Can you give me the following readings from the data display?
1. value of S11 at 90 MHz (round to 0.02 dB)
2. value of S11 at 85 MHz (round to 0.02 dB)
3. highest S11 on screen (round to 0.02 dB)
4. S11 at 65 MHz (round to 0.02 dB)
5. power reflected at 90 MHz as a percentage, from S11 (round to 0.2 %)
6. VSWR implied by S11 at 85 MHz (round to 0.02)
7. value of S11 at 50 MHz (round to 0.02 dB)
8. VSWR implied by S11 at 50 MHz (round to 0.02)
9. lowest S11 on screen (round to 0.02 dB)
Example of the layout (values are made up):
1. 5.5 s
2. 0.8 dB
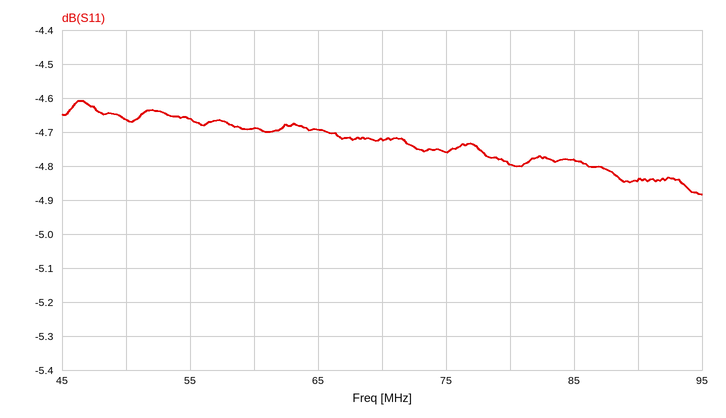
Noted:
1. -4.84 dB
2. -4.78 dB
3. -4.60 dB
4. -4.70 dB
5. 32.8 %
6. 3.72
7. -4.66 dB
8. 3.82
9. -4.88 dB
